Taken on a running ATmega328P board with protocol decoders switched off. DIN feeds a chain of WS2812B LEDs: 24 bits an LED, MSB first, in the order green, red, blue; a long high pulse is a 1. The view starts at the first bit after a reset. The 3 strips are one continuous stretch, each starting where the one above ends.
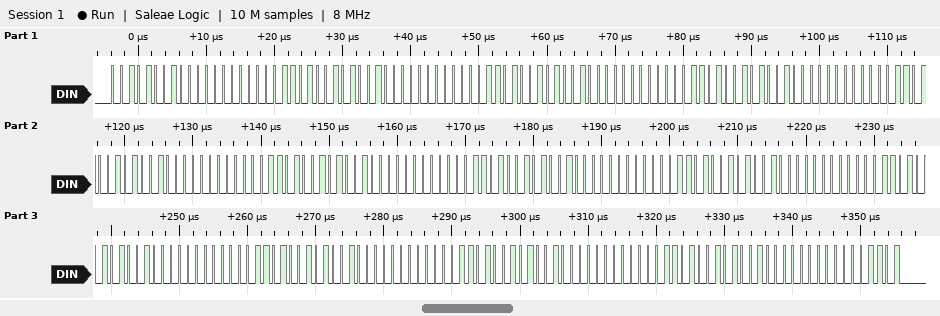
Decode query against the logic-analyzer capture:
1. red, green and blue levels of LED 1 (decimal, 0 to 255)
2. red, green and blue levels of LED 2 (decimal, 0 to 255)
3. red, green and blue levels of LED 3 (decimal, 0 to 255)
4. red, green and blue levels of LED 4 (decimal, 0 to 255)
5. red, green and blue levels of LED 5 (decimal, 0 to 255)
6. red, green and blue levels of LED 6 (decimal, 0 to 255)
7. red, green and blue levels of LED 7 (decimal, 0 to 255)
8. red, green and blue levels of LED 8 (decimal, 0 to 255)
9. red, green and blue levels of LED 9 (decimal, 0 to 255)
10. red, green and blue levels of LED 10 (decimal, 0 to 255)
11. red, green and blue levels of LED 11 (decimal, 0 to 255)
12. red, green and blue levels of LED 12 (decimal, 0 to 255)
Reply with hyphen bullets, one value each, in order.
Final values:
- 0, 41, 13
- 0, 41, 13
- 0, 41, 13
- 0, 41, 13
- 0, 41, 13
- 0, 41, 13
- 0, 41, 13
- 0, 41, 13
- 0, 41, 13
- 0, 41, 13
- 0, 41, 13
- 0, 41, 13
